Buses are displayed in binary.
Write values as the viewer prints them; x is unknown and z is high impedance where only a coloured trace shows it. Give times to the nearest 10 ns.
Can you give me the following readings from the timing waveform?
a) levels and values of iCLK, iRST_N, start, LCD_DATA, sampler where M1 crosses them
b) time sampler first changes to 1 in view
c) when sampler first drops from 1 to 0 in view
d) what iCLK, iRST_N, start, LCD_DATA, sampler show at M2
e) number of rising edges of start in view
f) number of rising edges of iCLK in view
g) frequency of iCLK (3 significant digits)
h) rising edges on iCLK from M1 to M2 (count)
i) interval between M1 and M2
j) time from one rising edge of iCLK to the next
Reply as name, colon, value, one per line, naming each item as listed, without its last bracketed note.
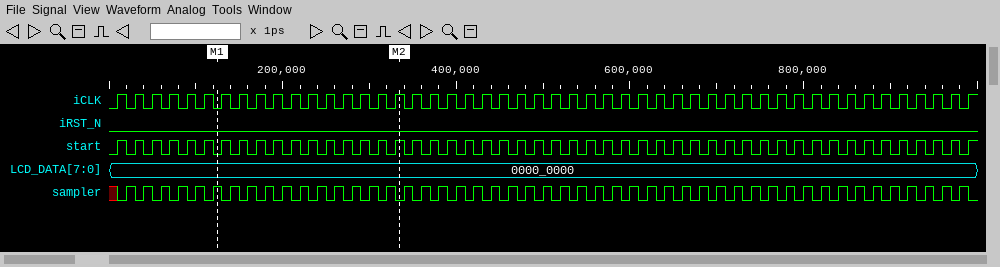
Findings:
levels and values of iCLK, iRST_N, start, LCD_DATA, sampler where M1 crosses them: iCLK=0, iRST_N=0, start=0, LCD_DATA=0000_0000, sampler=1
time sampler first changes to 1 in view: 20 ns
when sampler first drops from 1 to 0 in view: 30 ns
what iCLK, iRST_N, start, LCD_DATA, sampler show at M2: iCLK=1, iRST_N=0, start=1, LCD_DATA=0000_0000, sampler=0
number of rising edges of start in view: 50
number of rising edges of iCLK in view: 50
frequency of iCLK: 50.0 MHz
rising edges on iCLK from M1 to M2: 11
interval between M1 and M2: 210 ns
time from one rising edge of iCLK to the next: 20 ns
